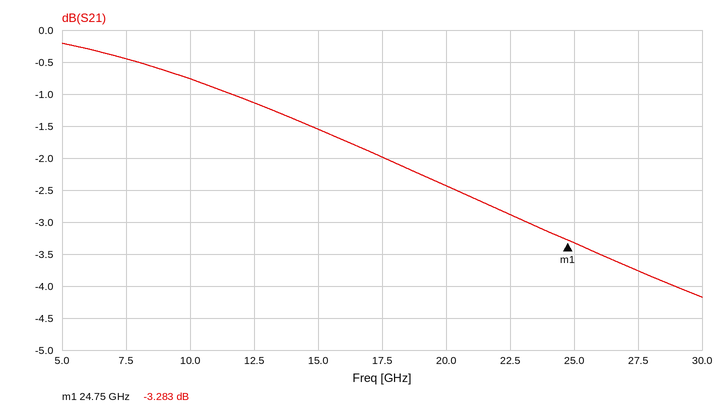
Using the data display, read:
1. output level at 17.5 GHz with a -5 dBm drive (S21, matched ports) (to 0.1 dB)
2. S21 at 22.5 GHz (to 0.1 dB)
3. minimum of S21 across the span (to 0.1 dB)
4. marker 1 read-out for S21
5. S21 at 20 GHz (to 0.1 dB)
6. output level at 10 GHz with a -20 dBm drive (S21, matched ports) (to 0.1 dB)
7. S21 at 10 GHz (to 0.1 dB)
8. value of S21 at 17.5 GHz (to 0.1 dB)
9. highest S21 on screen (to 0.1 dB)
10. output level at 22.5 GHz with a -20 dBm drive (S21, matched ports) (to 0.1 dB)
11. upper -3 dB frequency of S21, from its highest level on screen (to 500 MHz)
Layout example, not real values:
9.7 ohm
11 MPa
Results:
-7.0 dBm
-2.9 dB
-4.2 dB
-3.283 dB
-2.4 dB
-20.8 dBm
-0.8 dB
-2.0 dB
-0.2 dB
-22.9 dBm
24.5 GHz
